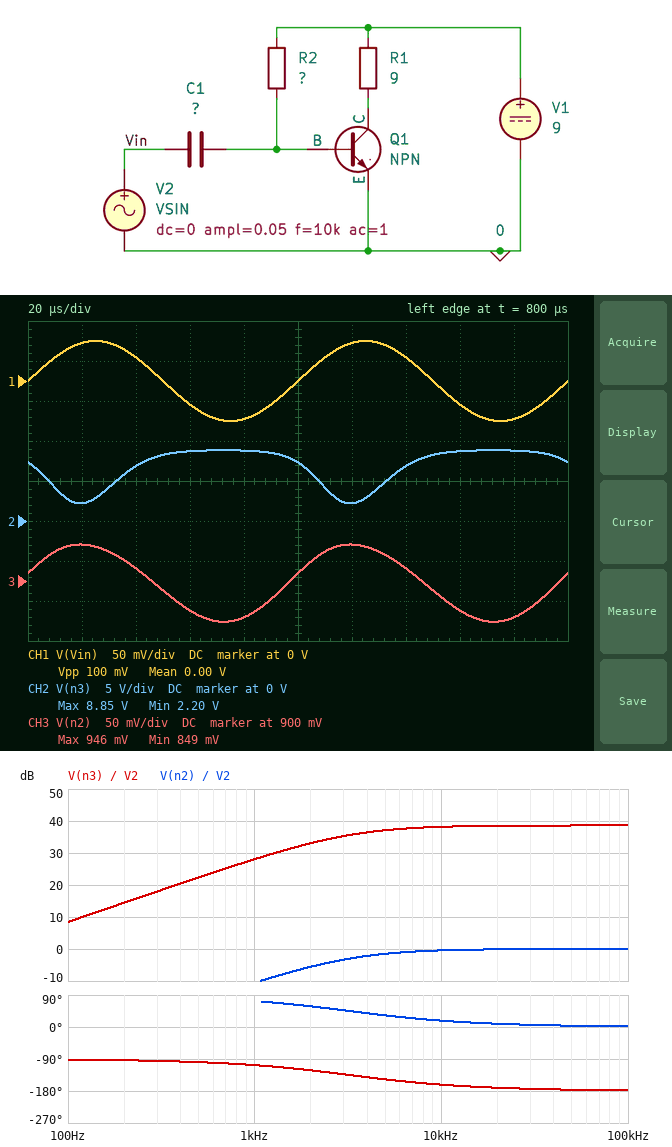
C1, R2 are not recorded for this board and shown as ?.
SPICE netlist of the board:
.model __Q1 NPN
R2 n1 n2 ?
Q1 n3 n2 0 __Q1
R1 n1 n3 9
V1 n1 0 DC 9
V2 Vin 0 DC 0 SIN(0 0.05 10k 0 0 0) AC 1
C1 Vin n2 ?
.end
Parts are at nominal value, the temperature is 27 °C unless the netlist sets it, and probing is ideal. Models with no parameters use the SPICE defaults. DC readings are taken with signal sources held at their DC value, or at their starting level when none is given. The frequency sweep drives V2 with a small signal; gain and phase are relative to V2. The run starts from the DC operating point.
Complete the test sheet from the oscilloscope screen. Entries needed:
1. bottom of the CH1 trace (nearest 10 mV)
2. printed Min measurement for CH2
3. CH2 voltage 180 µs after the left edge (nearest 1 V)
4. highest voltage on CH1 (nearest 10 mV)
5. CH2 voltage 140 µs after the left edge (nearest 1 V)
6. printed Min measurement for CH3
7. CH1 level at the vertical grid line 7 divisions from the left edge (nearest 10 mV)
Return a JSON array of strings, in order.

["-50 mV", "2.20 V", "9 V", "50 mV", "7 V", "849 mV", "30 mV"]
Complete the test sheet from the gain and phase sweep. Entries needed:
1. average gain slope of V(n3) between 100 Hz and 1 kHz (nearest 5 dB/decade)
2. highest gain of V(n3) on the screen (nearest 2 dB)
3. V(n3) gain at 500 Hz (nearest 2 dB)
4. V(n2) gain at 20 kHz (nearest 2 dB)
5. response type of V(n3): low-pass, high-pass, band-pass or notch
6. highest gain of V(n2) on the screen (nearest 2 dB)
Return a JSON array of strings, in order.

["20 dB/decade", "38 dB", "22 dB", "0 dB", "high-pass", "0 dB"]
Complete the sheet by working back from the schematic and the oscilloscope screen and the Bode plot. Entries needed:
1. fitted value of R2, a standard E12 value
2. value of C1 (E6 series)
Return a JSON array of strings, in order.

["3.3 kΩ", "4.7 µF"]
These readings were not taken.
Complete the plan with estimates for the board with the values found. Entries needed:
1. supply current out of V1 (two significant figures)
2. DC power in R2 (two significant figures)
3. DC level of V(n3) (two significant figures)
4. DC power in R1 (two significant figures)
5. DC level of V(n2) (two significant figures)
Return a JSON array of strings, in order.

["250 mA", "20 mW", "6.8 V", "540 mW", "920 mV"]
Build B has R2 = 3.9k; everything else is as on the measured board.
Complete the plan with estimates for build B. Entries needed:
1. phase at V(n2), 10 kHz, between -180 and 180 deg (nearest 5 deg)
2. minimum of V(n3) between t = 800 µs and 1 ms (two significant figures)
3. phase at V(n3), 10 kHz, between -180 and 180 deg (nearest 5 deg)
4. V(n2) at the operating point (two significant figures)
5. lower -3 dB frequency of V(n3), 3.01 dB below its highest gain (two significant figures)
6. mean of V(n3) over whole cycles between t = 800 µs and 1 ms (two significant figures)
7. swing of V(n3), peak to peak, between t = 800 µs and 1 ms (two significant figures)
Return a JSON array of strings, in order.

["15 deg", "3.2 V", "-165 deg", "910 mV", "2.7 kHz", "7.1 V", "5.7 V"]
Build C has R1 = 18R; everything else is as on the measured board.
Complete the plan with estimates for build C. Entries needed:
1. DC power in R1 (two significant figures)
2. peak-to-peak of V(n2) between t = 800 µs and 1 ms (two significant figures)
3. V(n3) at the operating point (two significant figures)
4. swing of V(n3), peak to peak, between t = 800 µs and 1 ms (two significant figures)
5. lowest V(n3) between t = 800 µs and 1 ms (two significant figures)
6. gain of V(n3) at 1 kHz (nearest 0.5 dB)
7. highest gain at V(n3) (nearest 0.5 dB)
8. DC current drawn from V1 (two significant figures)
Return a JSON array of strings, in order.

["1.1 W", "91 mV", "4.6 V", "8.6 V", "110 mV", "34.0 dB", "44.5 dB", "250 mA"]
